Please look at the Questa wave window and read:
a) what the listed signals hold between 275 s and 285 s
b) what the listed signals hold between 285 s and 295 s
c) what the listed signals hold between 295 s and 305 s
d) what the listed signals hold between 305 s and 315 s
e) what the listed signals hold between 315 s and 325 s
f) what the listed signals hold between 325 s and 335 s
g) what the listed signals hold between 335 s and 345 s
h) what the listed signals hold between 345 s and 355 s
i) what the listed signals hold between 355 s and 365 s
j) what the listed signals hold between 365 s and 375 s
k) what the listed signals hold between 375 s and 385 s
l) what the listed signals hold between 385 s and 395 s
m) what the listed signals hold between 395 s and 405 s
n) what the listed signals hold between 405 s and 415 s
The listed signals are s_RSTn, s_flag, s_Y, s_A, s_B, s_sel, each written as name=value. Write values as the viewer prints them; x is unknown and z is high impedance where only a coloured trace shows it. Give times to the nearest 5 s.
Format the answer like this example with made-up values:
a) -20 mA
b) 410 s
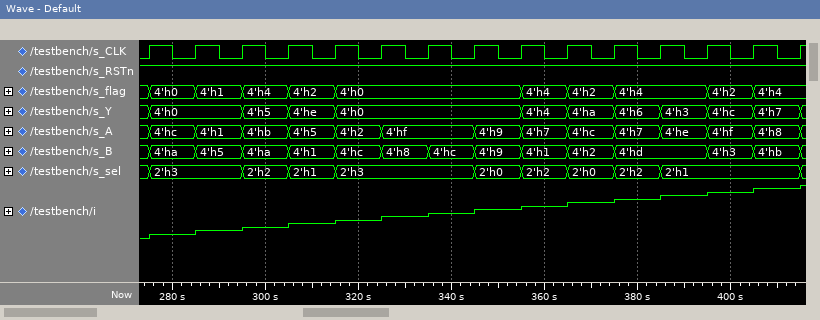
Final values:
a) s_RSTn=1, s_flag=4'h0, s_Y=4'h0, s_A=4'hc, s_B=4'ha, s_sel=2'h3
b) s_RSTn=1, s_flag=4'h1, s_Y=4'h0, s_A=4'h1, s_B=4'h5, s_sel=2'h3
c) s_RSTn=1, s_flag=4'h4, s_Y=4'h5, s_A=4'hb, s_B=4'ha, s_sel=2'h2
d) s_RSTn=1, s_flag=4'h2, s_Y=4'he, s_A=4'h5, s_B=4'h1, s_sel=2'h1
e) s_RSTn=1, s_flag=4'h0, s_Y=4'h0, s_A=4'h2, s_B=4'hc, s_sel=2'h3
f) s_RSTn=1, s_flag=4'h0, s_Y=4'h0, s_A=4'hf, s_B=4'h8, s_sel=2'h3
g) s_RSTn=1, s_flag=4'h0, s_Y=4'h0, s_A=4'hf, s_B=4'hc, s_sel=2'h3
h) s_RSTn=1, s_flag=4'h0, s_Y=4'h0, s_A=4'h9, s_B=4'h9, s_sel=2'h0
i) s_RSTn=1, s_flag=4'h4, s_Y=4'h4, s_A=4'h7, s_B=4'h1, s_sel=2'h2
j) s_RSTn=1, s_flag=4'h2, s_Y=4'ha, s_A=4'hc, s_B=4'h2, s_sel=2'h0
k) s_RSTn=1, s_flag=4'h4, s_Y=4'h6, s_A=4'h7, s_B=4'hd, s_sel=2'h2
l) s_RSTn=1, s_flag=4'h4, s_Y=4'h3, s_A=4'he, s_B=4'hd, s_sel=2'h1
m) s_RSTn=1, s_flag=4'h2, s_Y=4'hc, s_A=4'hf, s_B=4'h3, s_sel=2'h1
n) s_RSTn=1, s_flag=4'h4, s_Y=4'h7, s_A=4'h8, s_B=4'hb, s_sel=2'h1
